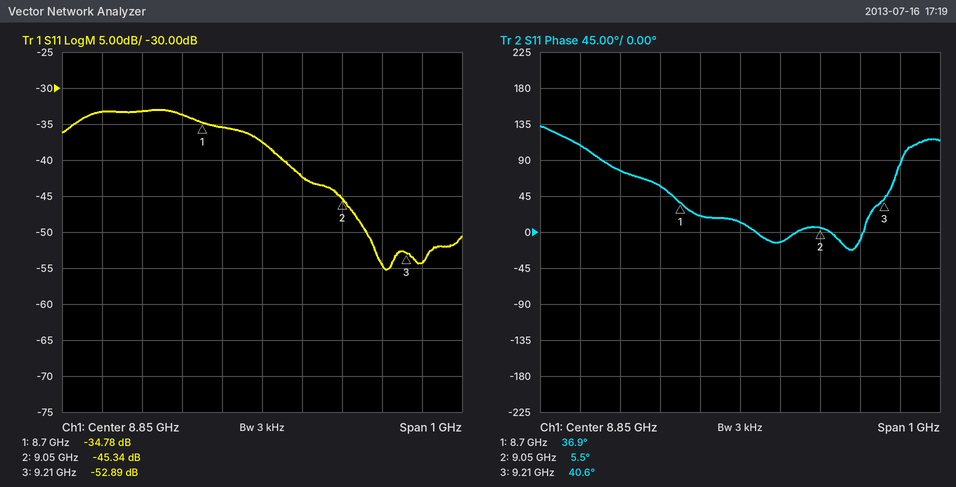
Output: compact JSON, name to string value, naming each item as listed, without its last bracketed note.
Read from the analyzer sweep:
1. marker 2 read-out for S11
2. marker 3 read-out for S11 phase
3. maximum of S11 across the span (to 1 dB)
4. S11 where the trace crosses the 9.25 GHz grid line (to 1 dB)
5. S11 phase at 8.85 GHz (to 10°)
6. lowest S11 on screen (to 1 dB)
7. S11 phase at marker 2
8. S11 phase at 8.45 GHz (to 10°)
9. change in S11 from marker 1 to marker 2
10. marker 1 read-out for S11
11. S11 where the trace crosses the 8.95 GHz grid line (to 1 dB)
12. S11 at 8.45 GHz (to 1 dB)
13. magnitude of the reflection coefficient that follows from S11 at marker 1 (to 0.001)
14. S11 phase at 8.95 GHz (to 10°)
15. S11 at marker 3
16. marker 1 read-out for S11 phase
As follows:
{"marker 2 read-out for S11": "-45.34 dB", "marker 3 read-out for S11 phase": "40.6°", "maximum of S11 across the span": "-33 dB", "S11 where the trace crosses the 9.25 GHz grid line": "-54 dB", "S11 phase at 8.85 GHz": "10°", "lowest S11 on screen": "-55 dB", "S11 phase at marker 2": "5.5°", "S11 phase at 8.45 GHz": "110°", "change in S11 from marker 1 to marker 2": "-10.56 dB", "marker 1 read-out for S11": "-34.78 dB", "S11 where the trace crosses the 8.95 GHz grid line": "-42 dB", "S11 at 8.45 GHz": "-33 dB", "magnitude of the reflection coefficient that follows from S11 at marker 1": "0.018", "S11 phase at 8.95 GHz": "-10°", "S11 at marker 3": "-52.89 dB", "marker 1 read-out for S11 phase": "36.9°"}
